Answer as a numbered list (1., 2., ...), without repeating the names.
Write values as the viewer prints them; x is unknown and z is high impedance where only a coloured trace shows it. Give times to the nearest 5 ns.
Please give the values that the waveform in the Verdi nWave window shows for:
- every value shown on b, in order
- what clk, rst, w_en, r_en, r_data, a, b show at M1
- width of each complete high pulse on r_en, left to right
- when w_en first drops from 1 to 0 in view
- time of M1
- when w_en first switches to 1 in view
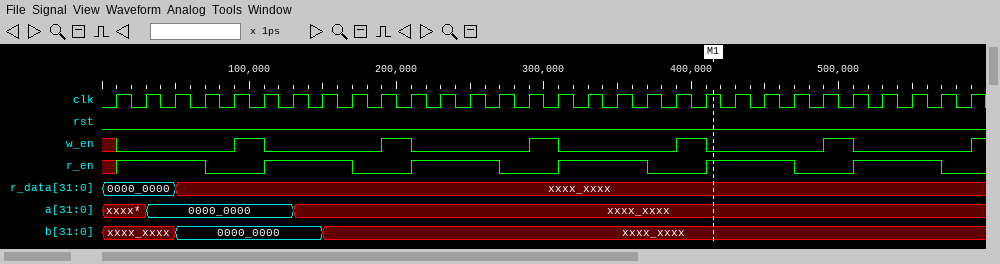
1. xxxx_xxxx, 0000_0000, xxxx_xxxx
2. clk=1, rst=0, w_en=0, r_en=1, r_data=xxxx_xxxx, a=xxxx_xxxx, b=xxxx_xxxx
3. 60 ns, 60 ns, 60 ns, 60 ns, 60 ns
4. 110 ns
5. 415 ns
6. 90 ns
